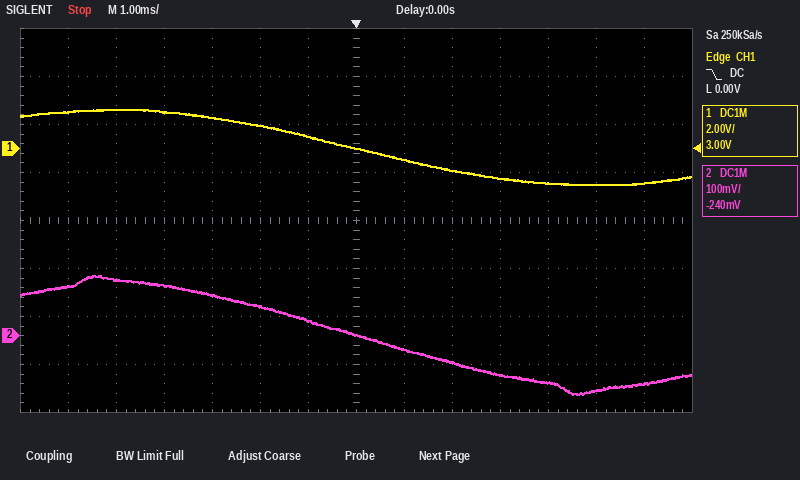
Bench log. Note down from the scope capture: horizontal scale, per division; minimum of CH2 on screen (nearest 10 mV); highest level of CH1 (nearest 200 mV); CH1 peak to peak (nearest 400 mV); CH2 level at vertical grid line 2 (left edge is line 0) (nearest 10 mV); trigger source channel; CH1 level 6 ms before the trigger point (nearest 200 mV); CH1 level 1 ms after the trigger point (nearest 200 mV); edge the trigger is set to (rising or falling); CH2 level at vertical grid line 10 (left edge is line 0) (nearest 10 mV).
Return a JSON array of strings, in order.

["1 ms", "-120 mV", "1.6 V", "3.2 V", "120 mV", "CH1", "1.6 V", "-400 mV", "falling", "-80 mV"]
